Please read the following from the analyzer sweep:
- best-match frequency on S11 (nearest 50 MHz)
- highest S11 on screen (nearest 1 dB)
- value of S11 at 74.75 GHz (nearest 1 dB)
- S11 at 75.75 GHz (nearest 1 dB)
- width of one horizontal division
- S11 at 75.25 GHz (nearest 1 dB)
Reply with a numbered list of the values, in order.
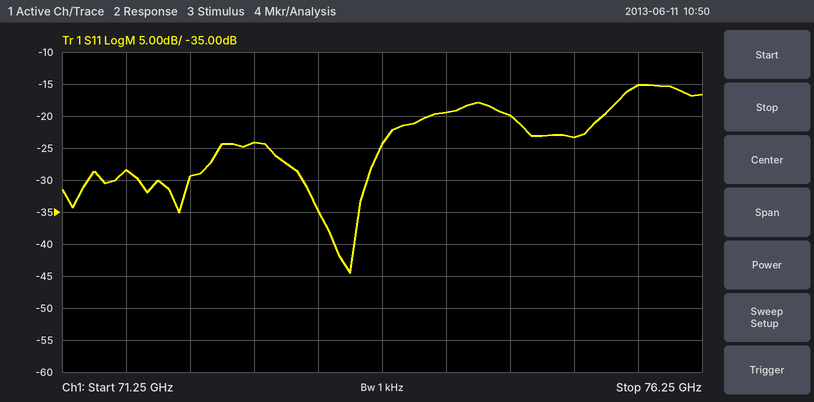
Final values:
1. 73.50 GHz
2. -15 dB
3. -20 dB
4. -15 dB
5. 500 MHz
6. -23 dB
